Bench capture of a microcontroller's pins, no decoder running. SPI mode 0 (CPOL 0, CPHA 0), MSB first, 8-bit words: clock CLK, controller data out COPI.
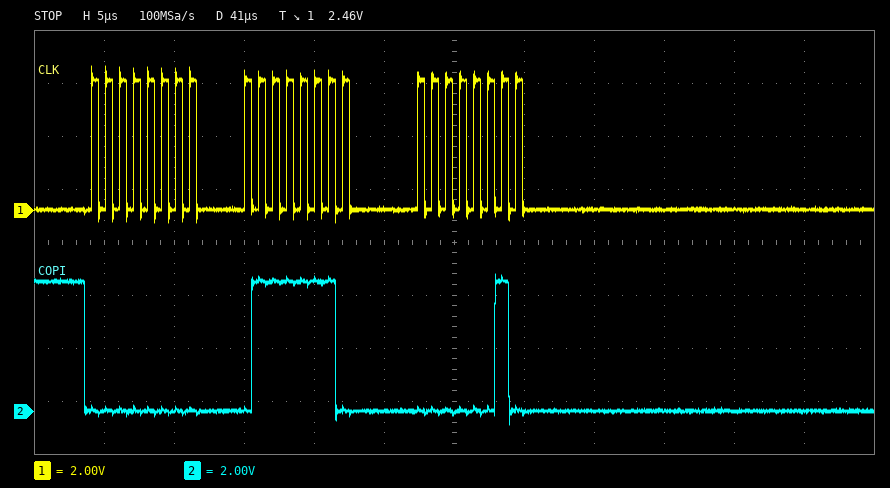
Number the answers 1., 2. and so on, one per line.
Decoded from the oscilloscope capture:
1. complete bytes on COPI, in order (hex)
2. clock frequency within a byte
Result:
1. 0x00 0x7E 0x02
2. 1 MHz
